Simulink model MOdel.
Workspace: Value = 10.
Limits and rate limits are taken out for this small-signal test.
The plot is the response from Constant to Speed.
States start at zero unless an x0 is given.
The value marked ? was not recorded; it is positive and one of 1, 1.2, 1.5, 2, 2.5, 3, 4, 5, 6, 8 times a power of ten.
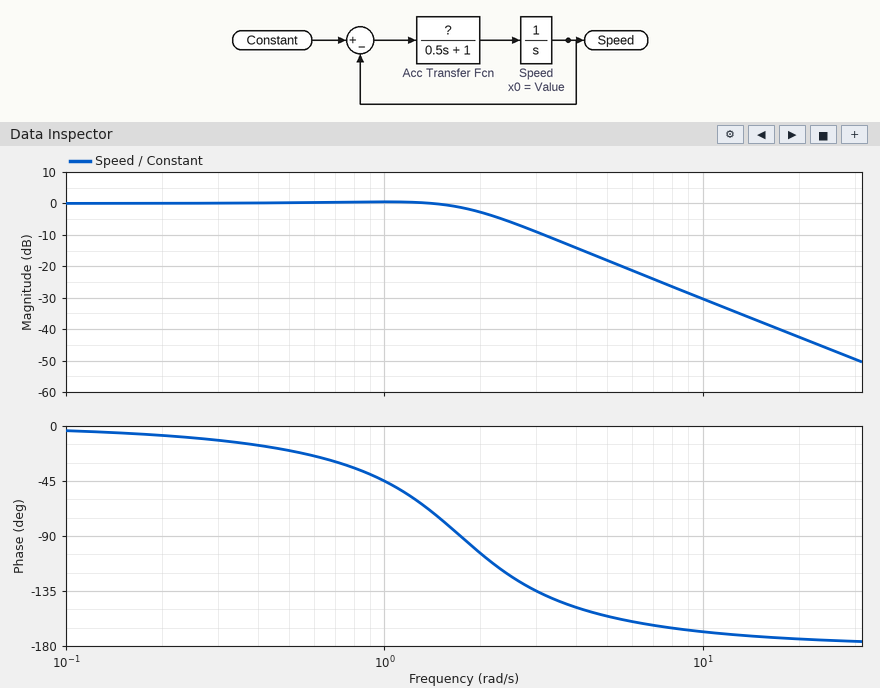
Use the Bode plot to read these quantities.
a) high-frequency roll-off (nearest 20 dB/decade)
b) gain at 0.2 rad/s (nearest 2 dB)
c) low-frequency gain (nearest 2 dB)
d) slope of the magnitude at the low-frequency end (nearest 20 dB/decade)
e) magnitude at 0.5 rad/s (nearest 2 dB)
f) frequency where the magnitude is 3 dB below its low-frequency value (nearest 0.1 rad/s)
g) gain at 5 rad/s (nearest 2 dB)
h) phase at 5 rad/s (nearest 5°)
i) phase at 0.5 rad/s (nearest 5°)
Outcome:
-40 dB/decade
0 dB
0 dB
0 dB/decade
0 dB
2.0 rad/s
-18 dB
-155°
-20°
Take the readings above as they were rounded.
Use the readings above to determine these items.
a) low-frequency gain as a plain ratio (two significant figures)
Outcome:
1.0
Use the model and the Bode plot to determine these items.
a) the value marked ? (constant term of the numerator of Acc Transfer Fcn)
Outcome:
1.5
